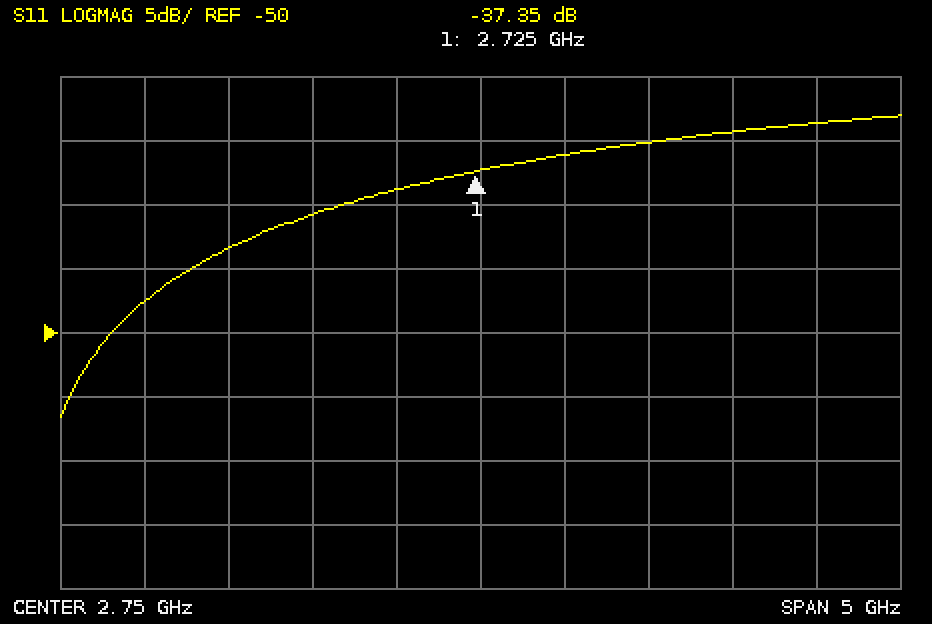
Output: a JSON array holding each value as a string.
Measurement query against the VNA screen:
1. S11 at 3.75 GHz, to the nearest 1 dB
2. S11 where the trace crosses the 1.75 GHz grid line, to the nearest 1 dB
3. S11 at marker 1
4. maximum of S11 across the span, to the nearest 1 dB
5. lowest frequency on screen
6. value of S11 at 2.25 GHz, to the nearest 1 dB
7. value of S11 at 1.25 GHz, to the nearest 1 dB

["-35 dB", "-41 dB", "-37.35 dB", "-33 dB", "250 MHz", "-39 dB", "-43 dB"]
